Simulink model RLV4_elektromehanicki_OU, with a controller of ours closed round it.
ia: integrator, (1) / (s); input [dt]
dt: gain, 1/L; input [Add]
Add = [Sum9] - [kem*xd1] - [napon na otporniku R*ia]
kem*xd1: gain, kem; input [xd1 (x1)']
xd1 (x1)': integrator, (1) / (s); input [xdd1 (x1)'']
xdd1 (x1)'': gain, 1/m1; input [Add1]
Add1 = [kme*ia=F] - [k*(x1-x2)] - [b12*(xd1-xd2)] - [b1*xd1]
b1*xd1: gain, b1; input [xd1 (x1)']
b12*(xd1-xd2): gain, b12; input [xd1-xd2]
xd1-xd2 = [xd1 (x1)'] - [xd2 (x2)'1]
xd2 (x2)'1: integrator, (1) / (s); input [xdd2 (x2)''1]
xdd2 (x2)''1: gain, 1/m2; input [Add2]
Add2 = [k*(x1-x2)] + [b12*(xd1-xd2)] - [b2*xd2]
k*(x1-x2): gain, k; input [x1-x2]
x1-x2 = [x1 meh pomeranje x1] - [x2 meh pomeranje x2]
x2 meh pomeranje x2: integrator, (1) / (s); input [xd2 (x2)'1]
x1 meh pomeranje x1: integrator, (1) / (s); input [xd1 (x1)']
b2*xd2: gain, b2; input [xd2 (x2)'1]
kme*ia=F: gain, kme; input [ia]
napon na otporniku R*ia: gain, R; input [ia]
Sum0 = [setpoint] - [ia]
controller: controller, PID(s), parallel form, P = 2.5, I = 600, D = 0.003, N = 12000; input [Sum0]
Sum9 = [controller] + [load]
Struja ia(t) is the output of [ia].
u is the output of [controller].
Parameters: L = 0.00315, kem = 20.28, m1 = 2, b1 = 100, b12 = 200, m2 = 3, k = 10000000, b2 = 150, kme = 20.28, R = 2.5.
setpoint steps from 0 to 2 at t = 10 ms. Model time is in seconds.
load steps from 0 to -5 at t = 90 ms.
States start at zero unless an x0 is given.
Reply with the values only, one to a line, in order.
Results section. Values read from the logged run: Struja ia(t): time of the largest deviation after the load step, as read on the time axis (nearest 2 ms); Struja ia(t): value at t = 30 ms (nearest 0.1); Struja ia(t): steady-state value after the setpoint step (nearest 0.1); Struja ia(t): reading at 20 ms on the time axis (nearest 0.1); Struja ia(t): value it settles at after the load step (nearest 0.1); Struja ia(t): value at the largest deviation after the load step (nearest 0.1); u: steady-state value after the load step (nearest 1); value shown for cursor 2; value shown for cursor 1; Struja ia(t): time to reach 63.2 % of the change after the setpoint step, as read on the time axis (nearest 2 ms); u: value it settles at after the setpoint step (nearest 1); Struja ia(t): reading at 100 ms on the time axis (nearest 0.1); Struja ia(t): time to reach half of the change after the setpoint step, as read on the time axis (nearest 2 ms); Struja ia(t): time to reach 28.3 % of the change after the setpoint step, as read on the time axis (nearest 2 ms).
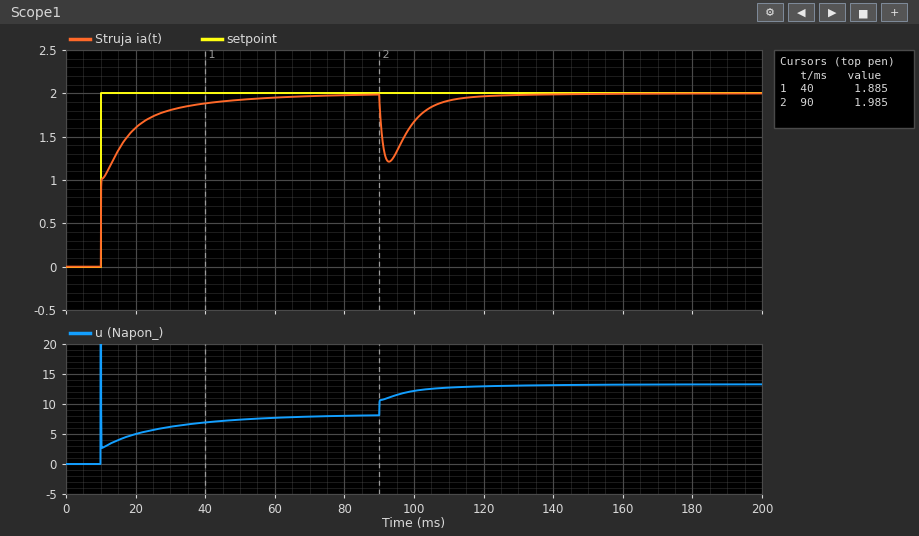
92 ms
1.8
2.0
1.6
2.0
1.2
13
1.985
1.885
14 ms
8
1.7
10 ms
10 ms
